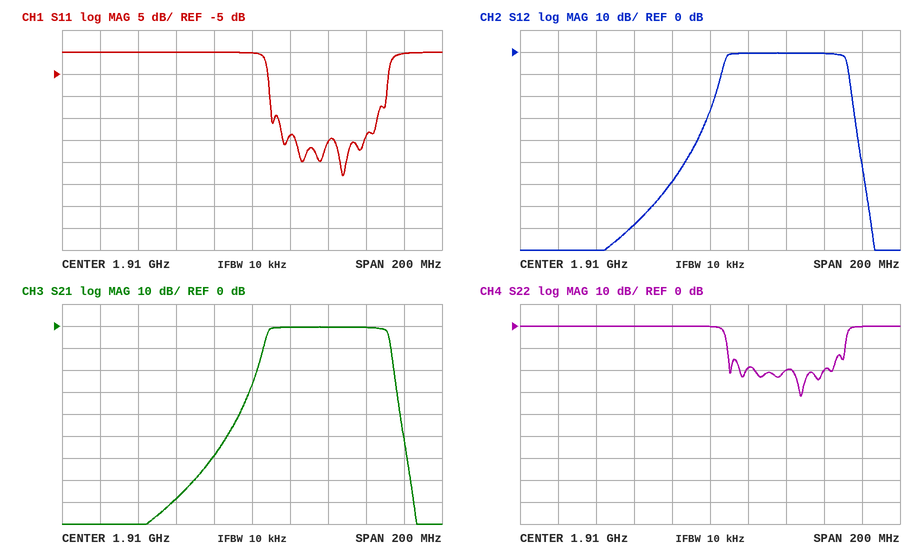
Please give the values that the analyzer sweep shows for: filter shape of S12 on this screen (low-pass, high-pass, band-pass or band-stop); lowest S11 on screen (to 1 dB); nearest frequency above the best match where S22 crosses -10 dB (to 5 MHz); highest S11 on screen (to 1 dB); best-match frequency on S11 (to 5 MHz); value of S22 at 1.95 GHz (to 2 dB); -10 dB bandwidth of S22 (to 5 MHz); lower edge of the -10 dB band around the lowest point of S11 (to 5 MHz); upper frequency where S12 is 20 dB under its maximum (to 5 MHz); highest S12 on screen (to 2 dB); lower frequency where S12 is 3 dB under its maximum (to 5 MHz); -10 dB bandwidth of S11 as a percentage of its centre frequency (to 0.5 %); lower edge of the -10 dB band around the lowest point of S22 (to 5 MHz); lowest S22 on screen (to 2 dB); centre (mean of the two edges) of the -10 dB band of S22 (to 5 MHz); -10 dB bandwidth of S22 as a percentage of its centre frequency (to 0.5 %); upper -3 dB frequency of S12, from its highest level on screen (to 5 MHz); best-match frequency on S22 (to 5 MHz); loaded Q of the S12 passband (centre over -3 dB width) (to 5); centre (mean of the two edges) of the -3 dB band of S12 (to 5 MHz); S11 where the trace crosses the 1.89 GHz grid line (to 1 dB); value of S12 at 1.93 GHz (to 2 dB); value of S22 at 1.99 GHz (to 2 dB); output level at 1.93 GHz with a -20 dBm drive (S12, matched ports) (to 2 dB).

band-pass
-28 dB
1.980 GHz
0 dB
1.960 GHz
-20 dB
60 MHz
1.920 GHz
1.985 GHz
0 dB
1.920 GHz
3.0 %
1.920 GHz
-32 dB
1.950 GHz
3.0 %
1.980 GHz
1.960 GHz
30
1.950 GHz
0 dB
0 dB
0 dB
-20 dBm
